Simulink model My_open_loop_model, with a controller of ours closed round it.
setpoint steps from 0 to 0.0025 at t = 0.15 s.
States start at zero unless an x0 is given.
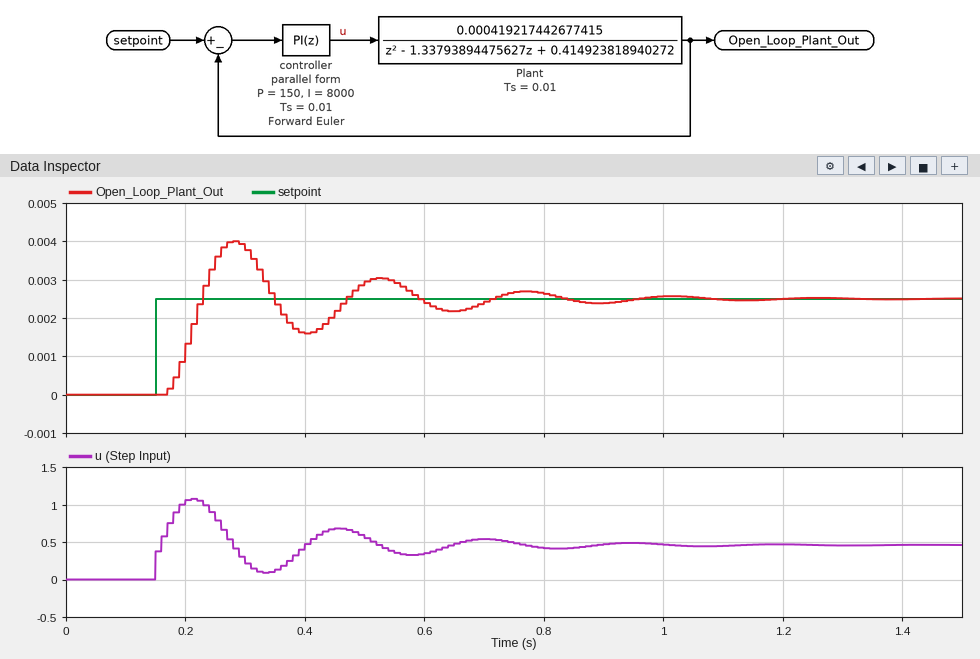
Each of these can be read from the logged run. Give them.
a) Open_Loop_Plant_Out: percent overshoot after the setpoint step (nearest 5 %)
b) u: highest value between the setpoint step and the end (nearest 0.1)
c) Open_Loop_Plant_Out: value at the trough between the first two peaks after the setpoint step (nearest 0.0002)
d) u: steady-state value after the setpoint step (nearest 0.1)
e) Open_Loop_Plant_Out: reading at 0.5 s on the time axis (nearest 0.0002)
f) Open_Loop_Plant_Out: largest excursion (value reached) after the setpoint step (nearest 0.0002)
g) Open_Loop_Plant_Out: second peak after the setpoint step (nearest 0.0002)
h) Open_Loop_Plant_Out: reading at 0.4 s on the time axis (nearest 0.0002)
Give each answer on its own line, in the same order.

60 %
1.1
0.0016
0.5
0.0030
0.0040
0.0030
0.0016
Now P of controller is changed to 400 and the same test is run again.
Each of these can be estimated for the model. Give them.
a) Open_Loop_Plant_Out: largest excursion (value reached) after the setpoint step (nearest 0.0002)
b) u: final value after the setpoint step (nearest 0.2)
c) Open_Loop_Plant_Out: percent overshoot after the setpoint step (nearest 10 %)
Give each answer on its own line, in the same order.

0.0034
0.4
30 %
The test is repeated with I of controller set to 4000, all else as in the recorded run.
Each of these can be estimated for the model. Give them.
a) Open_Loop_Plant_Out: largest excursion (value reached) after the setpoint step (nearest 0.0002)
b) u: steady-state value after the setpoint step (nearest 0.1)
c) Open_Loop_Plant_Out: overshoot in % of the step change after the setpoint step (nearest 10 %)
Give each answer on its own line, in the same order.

0.0030
0.5
20 %
